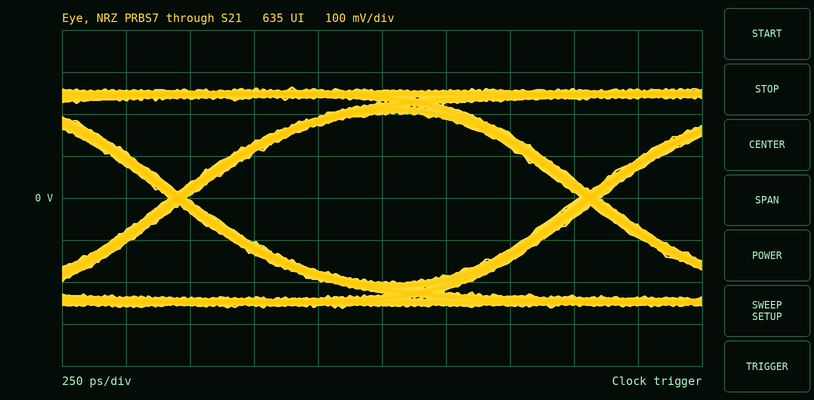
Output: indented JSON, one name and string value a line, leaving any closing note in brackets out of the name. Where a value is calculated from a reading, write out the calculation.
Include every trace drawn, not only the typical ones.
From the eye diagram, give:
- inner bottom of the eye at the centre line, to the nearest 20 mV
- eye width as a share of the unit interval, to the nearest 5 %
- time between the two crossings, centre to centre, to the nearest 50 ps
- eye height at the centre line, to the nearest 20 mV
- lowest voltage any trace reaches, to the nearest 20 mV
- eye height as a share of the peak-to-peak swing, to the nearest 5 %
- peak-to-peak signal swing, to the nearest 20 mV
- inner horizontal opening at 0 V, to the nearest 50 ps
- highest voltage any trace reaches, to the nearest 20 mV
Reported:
{
  "inner bottom of the eye at the centre line, to the nearest 20 mV": "-200 mV",
  "eye width as a share of the unit interval, to the nearest 5 %": "1.55 ns / 1.60 ns ≈ 96.9 %, so 95 % to the nearest 5 %",
  "time between the two crossings, centre to centre, to the nearest 50 ps": "1.60 ns",
  "eye height at the centre line, to the nearest 20 mV": "400 mV",
  "lowest voltage any trace reaches, to the nearest 20 mV": "-260 mV",
  "eye height as a share of the peak-to-peak swing, to the nearest 5 %": "400 mV / 520 mV ≈ 76.9 %, so 75 % to the nearest 5 %",
  "peak-to-peak signal swing, to the nearest 20 mV": "520 mV",
  "inner horizontal opening at 0 V, to the nearest 50 ps": "1.55 ns",
  "highest voltage any trace reaches, to the nearest 20 mV": "260 mV"
}
